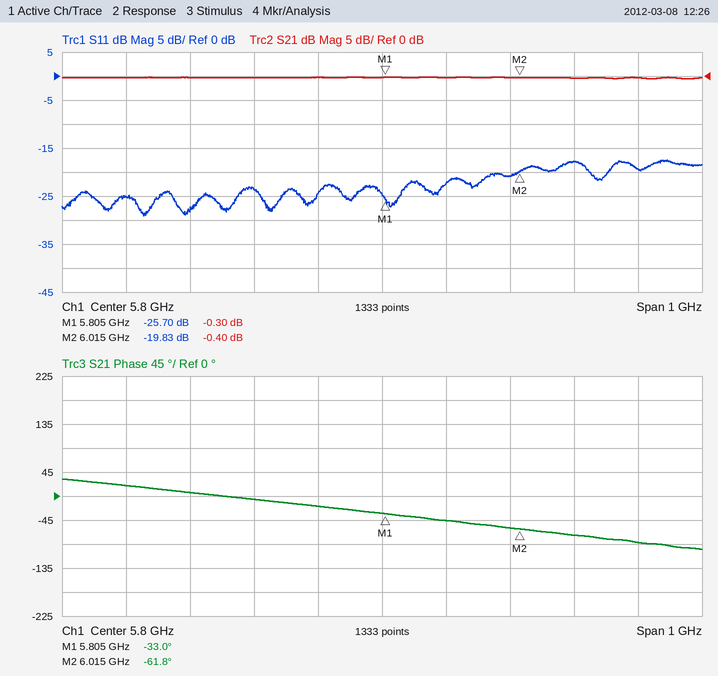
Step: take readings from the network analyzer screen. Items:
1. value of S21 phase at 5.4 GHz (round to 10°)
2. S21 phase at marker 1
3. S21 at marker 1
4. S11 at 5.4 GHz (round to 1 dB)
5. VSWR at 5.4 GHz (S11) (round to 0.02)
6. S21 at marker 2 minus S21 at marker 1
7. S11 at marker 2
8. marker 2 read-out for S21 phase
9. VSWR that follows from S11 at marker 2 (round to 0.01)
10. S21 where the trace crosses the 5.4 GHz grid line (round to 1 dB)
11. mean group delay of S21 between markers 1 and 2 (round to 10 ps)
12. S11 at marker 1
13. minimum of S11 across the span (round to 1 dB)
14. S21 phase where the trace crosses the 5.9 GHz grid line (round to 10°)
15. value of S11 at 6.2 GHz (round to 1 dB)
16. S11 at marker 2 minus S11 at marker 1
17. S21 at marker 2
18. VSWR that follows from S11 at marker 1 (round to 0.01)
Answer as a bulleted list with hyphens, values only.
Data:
- 20°
- -33.0°
- -0.30 dB
- -25 dB
- 1.12
- -0.10 dB
- -19.83 dB
- -61.8°
- 1.23
- 0 dB
- 380 ps
- -25.70 dB
- -29 dB
- -50°
- -19 dB
- 5.87 dB
- -0.40 dB
- 1.11
